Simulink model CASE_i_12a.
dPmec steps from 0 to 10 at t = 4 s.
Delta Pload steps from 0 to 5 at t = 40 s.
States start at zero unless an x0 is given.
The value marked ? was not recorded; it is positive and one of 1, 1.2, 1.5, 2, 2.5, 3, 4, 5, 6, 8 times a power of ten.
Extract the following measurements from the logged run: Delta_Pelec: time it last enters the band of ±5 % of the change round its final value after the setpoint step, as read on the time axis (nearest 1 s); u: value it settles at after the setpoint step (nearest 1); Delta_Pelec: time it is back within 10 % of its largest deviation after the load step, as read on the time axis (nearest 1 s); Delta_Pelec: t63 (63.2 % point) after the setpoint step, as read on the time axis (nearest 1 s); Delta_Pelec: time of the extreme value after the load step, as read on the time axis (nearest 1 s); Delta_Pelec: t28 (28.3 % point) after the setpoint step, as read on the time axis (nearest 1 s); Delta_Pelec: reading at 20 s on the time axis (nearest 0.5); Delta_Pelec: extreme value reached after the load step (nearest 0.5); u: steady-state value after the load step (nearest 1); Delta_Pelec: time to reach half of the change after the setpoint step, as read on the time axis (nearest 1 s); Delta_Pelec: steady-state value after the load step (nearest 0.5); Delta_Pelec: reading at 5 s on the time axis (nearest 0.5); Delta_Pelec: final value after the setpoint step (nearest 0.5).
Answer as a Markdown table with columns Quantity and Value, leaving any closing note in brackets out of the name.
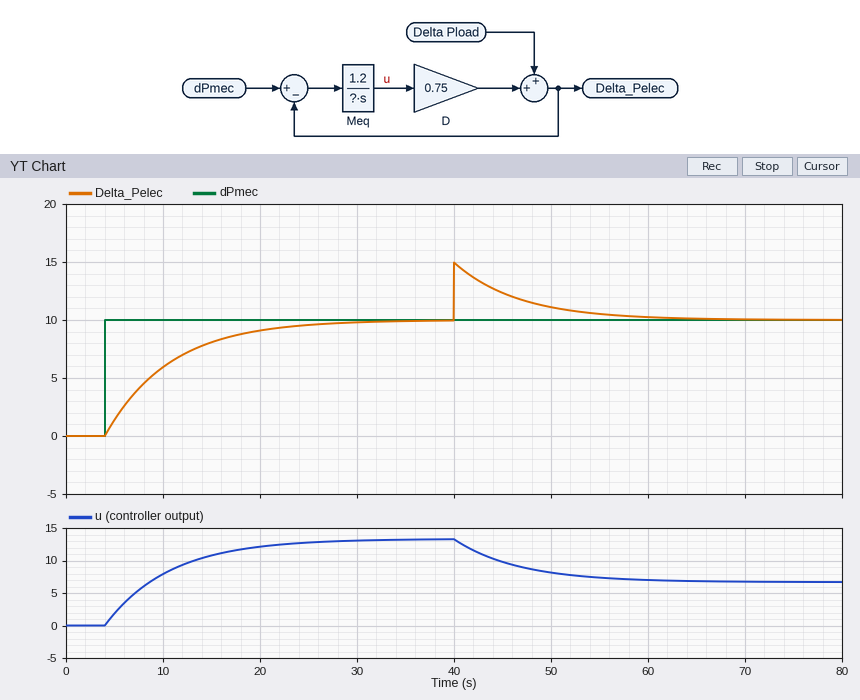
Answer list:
| Quantity | Value |
|---|---|
| Delta_Pelec: time it last enters the band of ±5 % of the change round its final value after the setpoint step, as read on the time axis | 24 s |
| u: value it settles at after the setpoint step | 13 |
| Delta_Pelec: time it is back within 10 % of its largest deviation after the load step, as read on the time axis | 55 s |
| Delta_Pelec: t63 (63.2 % point) after the setpoint step, as read on the time axis | 11 s |
| Delta_Pelec: time of the extreme value after the load step, as read on the time axis | 40 s |
| Delta_Pelec: t28 (28.3 % point) after the setpoint step, as read on the time axis | 6 s |
| Delta_Pelec: reading at 20 s on the time axis | 9.0 |
| Delta_Pelec: extreme value reached after the load step | 15.0 |
| u: steady-state value after the load step | 7 |
| Delta_Pelec: time to reach half of the change after the setpoint step, as read on the time axis | 9 s |
| Delta_Pelec: steady-state value after the load step | 10.0 |
| Delta_Pelec: reading at 5 s on the time axis | 1.5 |
| Delta_Pelec: final value after the setpoint step | 10.0 |
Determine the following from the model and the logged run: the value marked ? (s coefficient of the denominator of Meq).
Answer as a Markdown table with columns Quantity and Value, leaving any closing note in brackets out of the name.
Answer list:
| Quantity | Value |
|---|---|
| the value marked ? | 6 |
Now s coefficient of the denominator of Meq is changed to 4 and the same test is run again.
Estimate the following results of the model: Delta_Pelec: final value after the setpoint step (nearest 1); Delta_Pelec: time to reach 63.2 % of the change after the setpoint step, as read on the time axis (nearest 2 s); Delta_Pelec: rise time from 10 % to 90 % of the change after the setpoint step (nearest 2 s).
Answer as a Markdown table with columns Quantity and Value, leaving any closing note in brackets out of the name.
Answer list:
| Quantity | Value |
|---|---|
| Delta_Pelec: final value after the setpoint step | 10 |
| Delta_Pelec: time to reach 63.2 % of the change after the setpoint step, as read on the time axis | 8 s |
| Delta_Pelec: rise time from 10 % to 90 % of the change after the setpoint step | 10 s |
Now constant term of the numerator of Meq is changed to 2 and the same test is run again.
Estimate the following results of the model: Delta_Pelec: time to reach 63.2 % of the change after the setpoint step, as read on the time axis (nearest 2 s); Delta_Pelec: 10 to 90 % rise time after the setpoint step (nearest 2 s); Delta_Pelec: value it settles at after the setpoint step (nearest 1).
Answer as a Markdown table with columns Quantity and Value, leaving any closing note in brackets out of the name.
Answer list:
| Quantity | Value |
|---|---|
| Delta_Pelec: time to reach 63.2 % of the change after the setpoint step, as read on the time axis | 8 s |
| Delta_Pelec: 10 to 90 % rise time after the setpoint step | 8 s |
| Delta_Pelec: value it settles at after the setpoint step | 10 |
